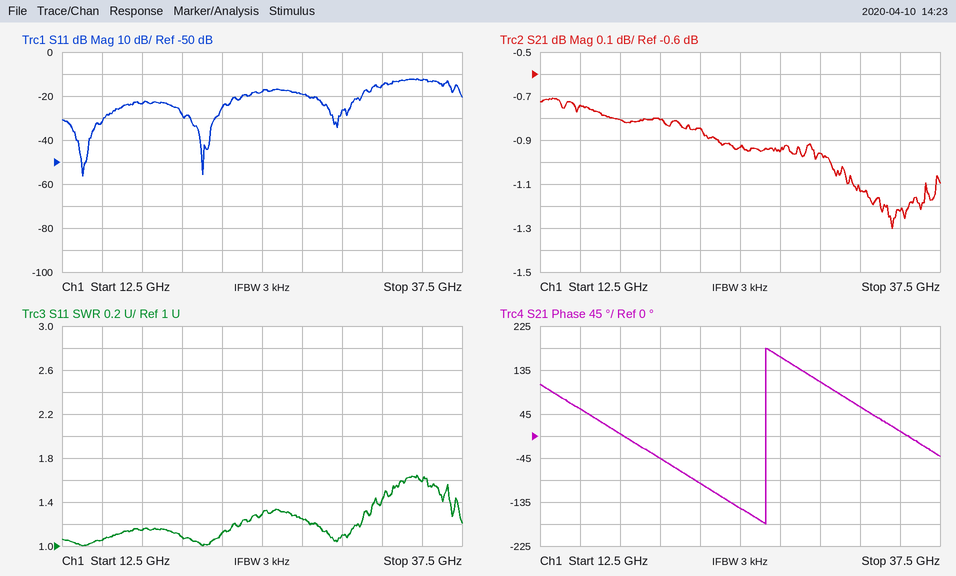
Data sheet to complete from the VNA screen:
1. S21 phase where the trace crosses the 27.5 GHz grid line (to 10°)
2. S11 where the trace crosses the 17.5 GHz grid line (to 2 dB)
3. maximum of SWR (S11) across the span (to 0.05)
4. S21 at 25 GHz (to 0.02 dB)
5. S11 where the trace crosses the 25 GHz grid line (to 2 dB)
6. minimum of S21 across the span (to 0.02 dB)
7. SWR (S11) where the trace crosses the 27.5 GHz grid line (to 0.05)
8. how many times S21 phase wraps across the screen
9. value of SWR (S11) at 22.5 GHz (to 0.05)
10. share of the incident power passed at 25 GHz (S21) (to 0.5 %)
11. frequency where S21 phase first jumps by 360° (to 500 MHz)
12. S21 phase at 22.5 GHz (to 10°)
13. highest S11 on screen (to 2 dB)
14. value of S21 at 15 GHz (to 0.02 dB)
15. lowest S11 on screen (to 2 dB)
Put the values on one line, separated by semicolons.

160°; -24 dB; 1.65; -0.94 dB; -18 dB; -1.30 dB; 1.25; 1; 1.10; 80.5 %; 26.5 GHz; -100°; -12 dB; -0.74 dB; -56 dB
